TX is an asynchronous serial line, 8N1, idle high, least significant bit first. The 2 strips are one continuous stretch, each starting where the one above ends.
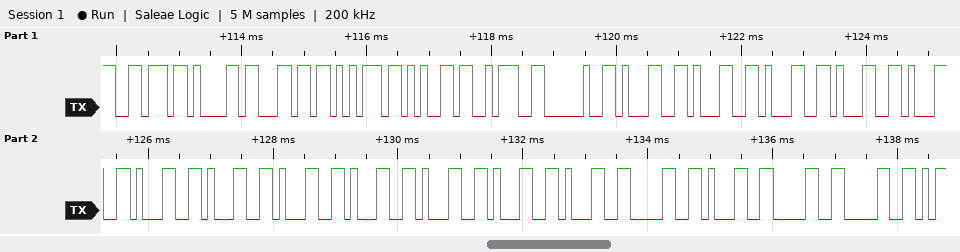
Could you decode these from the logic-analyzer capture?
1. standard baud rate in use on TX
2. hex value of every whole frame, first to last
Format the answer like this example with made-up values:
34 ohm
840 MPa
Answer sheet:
9600 baud
0x76 0x61 0x6C 0x75 0x65 0x3A 0x20 0x31 0x31 0x31 0x31 0x31 0x31 0x31 0x31 0x31 0x31 0x31 0x31 0x30 0x31 0x30 0x30
